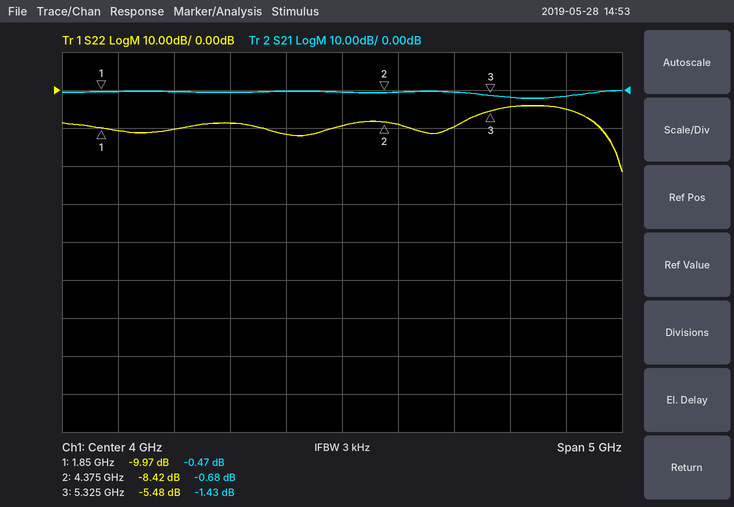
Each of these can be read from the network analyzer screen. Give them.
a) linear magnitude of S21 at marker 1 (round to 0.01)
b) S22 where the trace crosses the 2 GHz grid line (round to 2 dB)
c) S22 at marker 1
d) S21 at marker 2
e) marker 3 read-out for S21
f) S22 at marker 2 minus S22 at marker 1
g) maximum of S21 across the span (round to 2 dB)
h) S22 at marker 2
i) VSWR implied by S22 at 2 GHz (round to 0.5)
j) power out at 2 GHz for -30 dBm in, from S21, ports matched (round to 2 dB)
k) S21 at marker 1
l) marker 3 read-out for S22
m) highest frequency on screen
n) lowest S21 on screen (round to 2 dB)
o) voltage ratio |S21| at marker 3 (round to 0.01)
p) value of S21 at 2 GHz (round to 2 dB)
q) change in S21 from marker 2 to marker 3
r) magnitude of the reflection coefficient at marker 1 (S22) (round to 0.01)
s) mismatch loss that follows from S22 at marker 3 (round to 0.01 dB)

0.95
-10 dB
-9.97 dB
-0.68 dB
-1.43 dB
1.55 dB
0 dB
-8.42 dB
2.0
-30 dBm
-0.47 dB
-5.48 dB
6.5 GHz
-2 dB
0.85
0 dB
-0.75 dB
0.32
1.45 dB
